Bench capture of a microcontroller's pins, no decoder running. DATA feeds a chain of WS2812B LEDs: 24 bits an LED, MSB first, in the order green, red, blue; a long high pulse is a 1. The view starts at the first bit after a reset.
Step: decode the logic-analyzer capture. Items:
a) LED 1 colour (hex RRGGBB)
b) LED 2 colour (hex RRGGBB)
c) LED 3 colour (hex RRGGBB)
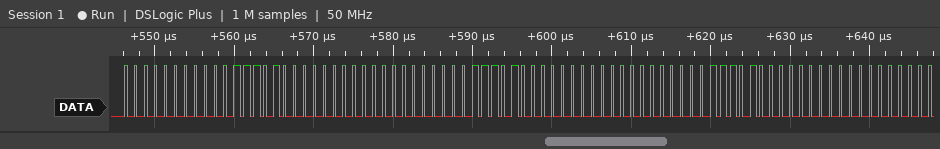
#1D0000
#1D0000
#1D0000
